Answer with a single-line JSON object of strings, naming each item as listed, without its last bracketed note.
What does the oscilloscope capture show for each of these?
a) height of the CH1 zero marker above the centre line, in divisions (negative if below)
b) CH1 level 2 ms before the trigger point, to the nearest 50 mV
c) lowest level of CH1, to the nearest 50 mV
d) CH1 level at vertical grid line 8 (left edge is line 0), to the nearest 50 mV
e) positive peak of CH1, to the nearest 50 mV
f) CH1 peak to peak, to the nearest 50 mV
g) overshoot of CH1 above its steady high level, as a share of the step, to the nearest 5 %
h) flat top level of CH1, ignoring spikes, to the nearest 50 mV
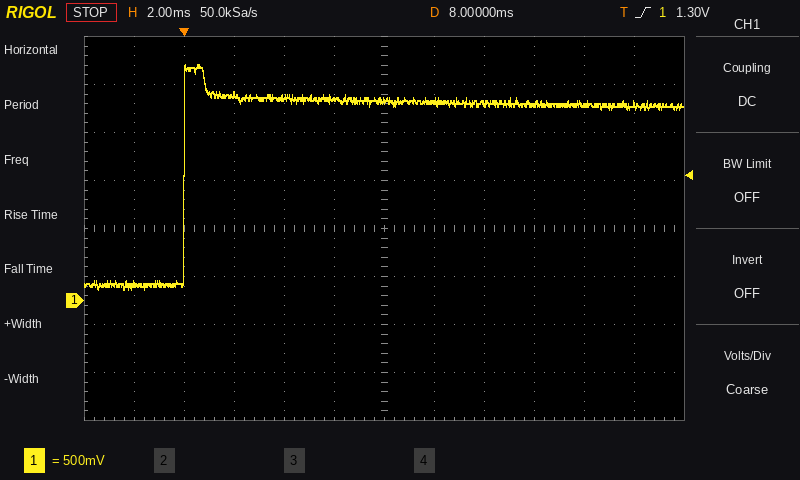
{"height of the CH1 zero marker above the centre line, in divisions": "-1.5 div", "CH1 level 2 ms before the trigger point, to the nearest 50 mV": "150 mV", "lowest level of CH1, to the nearest 50 mV": "100 mV", "CH1 level at vertical grid line 8 (left edge is line 0), to the nearest 50 mV": "2.05 V", "positive peak of CH1, to the nearest 50 mV": "2.45 V", "CH1 peak to peak, to the nearest 50 mV": "2.35 V", "overshoot of CH1 above its steady high level, as a share of the step, to the nearest 5 %": "20 %", "flat top level of CH1, ignoring spikes, to the nearest 50 mV": "2.05 V"}
